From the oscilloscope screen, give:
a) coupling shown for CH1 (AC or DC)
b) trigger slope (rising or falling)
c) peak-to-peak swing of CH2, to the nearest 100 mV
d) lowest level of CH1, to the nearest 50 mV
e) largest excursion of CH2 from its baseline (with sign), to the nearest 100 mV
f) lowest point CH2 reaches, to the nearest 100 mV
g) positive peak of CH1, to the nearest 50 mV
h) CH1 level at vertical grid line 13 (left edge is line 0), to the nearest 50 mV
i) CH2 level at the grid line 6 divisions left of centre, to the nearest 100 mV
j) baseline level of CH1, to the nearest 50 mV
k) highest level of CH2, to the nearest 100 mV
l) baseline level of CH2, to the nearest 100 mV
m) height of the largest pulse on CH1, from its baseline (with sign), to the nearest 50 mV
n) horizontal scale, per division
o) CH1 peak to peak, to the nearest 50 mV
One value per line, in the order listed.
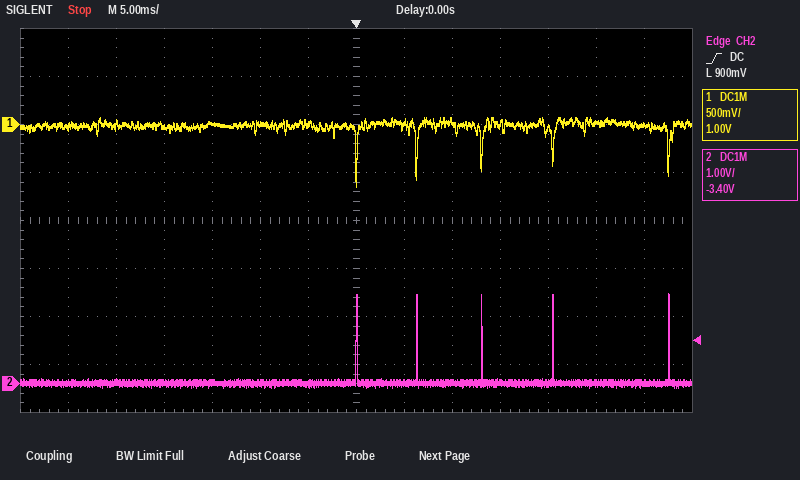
DC
rising
2.0 V
-650 mV
+1.9 V
-100 mV
50 mV
0 mV
0.0 V
0 mV
1.9 V
0.0 V
-650 mV
5 ms
700 mV
